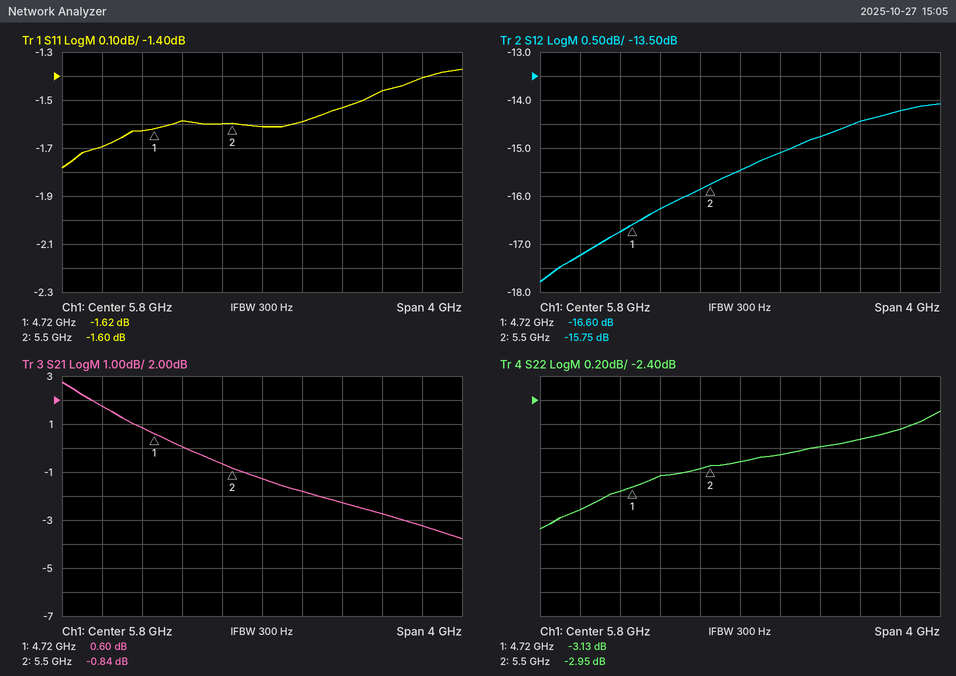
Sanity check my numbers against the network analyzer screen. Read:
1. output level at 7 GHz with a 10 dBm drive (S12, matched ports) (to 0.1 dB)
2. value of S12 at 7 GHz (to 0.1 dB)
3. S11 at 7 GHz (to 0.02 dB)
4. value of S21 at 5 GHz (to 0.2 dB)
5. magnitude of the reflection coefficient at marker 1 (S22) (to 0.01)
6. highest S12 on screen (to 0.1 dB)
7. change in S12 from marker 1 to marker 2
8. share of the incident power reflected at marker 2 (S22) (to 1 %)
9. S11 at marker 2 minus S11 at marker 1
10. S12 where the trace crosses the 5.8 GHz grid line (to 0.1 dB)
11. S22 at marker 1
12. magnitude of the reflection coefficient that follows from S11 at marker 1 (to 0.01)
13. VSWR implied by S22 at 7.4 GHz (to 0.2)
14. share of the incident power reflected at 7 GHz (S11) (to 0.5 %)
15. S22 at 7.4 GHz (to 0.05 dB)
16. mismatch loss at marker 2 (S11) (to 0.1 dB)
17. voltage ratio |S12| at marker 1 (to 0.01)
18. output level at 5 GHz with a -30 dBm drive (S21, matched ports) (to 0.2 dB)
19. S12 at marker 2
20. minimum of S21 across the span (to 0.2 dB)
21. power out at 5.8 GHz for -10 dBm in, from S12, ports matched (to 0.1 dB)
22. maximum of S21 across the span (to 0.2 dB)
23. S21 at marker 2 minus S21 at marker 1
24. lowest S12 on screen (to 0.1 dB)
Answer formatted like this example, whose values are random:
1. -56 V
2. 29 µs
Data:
1. -4.4 dBm
2. -14.4 dB
3. -1.46 dB
4. 0.0 dB
5. 0.70
6. -14.1 dB
7. 0.85 dB
8. 51 %
9. 0.02 dB
10. -15.5 dB
11. -3.13 dB
12. 0.83
13. 6.6
14. 71.5 %
15. -2.65 dB
16. 5.1 dB
17. 0.15
18. -30.0 dBm
19. -15.75 dB
20. -3.8 dB
21. -25.5 dBm
22. 2.8 dB
23. -1.44 dB
24. -17.8 dB
